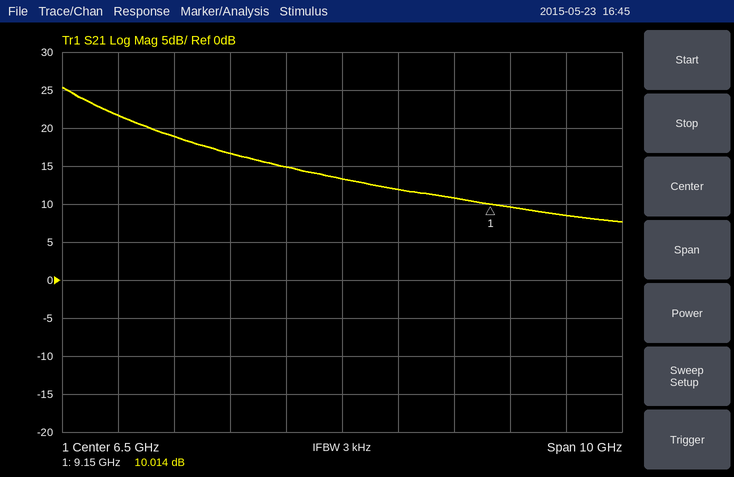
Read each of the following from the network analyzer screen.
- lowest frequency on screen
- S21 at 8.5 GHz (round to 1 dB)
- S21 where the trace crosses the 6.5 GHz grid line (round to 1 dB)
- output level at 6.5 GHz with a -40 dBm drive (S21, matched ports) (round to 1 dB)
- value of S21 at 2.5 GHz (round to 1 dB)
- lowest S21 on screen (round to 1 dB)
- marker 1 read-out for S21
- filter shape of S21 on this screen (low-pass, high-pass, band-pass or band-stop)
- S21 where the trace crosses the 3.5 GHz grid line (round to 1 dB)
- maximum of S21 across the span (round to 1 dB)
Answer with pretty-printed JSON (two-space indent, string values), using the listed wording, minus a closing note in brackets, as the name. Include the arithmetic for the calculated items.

{
  "lowest frequency on screen": "1.5 GHz",
  "S21 at 8.5 GHz": "11 dB",
  "S21 where the trace crosses the 6.5 GHz grid line": "13 dB",
  "output level at 6.5 GHz with a -40 dBm drive (S21, matched ports)": "-40 dBm + (13 dB) = -27 dBm",
  "value of S21 at 2.5 GHz": "22 dB",
  "lowest S21 on screen": "8 dB",
  "marker 1 read-out for S21": "10.014 dB",
  "filter shape of S21 on this screen": "low-pass",
  "S21 where the trace crosses the 3.5 GHz grid line": "19 dB",
  "maximum of S21 across the span": "25 dB"
}
